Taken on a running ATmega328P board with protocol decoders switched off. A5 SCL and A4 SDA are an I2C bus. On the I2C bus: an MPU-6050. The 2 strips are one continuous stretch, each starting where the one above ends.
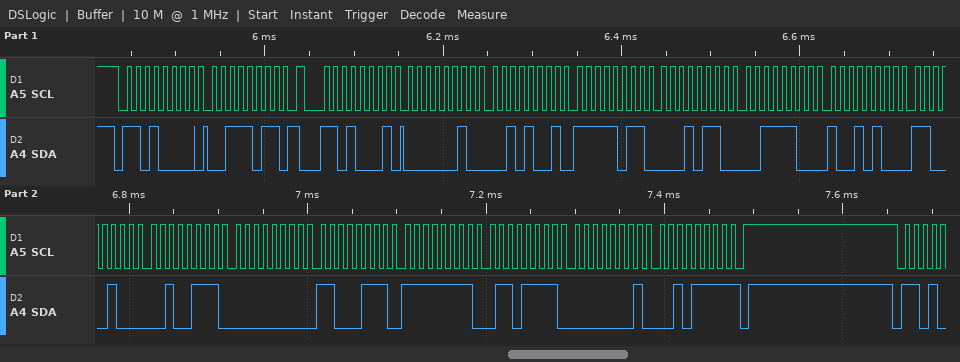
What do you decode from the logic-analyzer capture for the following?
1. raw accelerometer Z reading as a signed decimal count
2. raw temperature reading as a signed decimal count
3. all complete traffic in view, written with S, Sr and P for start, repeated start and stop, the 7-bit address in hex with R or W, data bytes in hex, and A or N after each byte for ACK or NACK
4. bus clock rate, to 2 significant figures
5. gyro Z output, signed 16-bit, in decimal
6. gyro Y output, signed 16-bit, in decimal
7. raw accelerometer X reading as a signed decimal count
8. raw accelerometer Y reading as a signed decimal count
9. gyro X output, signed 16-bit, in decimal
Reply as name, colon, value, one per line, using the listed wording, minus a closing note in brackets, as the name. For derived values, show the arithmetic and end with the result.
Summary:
raw accelerometer Z reading as a signed decimal count: 0x3C94 = 15508
raw temperature reading as a signed decimal count: 0xC427 = -15321
all complete traffic in view, written with S, Sr and P for start, repeated start and stop, the 7-bit address in hex with R or W, data bytes in hex, and A or N after each byte for ACK or NACK: S 68W A 3B A Sr 68R A 02 A 29 A FB A 16 A 3C A 94 A C4 A 27 A 00 A C7 A FF A 6F A 01 A 2F N P
bus clock rate, to 2 significant figures: 100 kHz
gyro Z output, signed 16-bit, in decimal: 0x012F = 303
gyro Y output, signed 16-bit, in decimal: 0xFF6F = -145
raw accelerometer X reading as a signed decimal count: 0x0229 = 553
raw accelerometer Y reading as a signed decimal count: 0xFB16 = -1258
gyro X output, signed 16-bit, in decimal: 0x00C7 = 199
